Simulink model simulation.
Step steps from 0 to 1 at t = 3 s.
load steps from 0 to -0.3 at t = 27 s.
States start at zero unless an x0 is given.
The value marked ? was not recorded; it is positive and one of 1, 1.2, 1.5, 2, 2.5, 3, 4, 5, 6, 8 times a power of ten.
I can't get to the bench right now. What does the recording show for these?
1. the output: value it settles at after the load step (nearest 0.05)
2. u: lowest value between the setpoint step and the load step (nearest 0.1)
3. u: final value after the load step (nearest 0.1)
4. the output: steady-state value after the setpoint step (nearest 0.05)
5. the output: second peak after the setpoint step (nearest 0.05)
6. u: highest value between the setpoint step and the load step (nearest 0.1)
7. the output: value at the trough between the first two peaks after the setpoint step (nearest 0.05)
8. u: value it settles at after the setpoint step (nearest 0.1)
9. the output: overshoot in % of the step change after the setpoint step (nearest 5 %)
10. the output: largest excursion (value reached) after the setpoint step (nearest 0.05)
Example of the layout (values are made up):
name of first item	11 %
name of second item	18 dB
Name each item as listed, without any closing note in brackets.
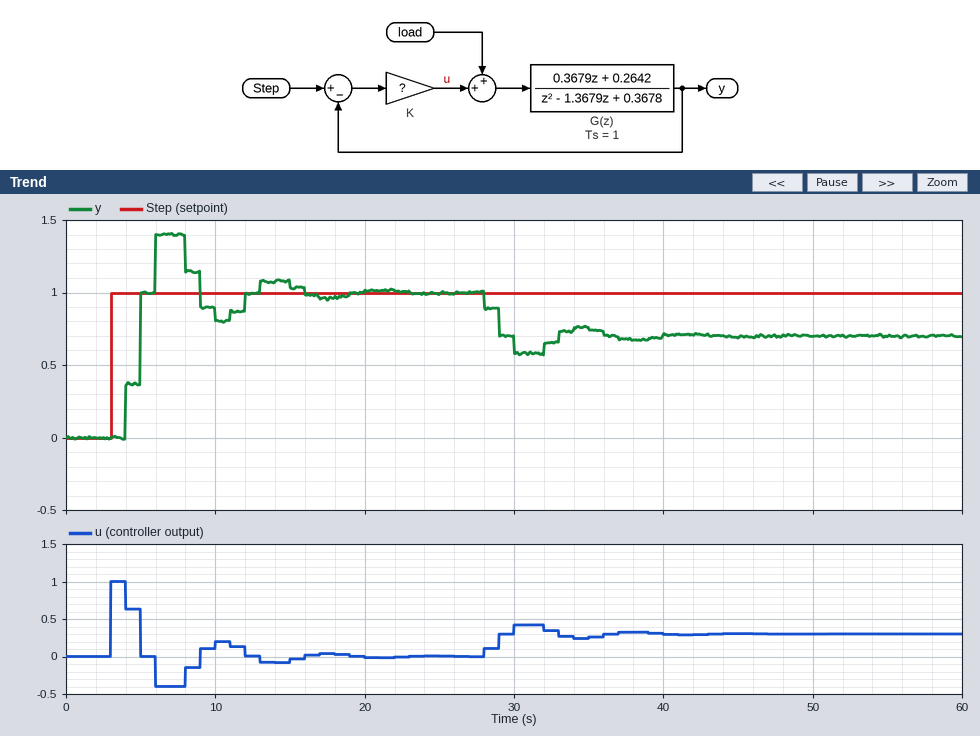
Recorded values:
the output: value it settles at after the load step	0.70
u: lowest value between the setpoint step and the load step	-0.4
u: final value after the load step	0.3
the output: steady-state value after the setpoint step	1.00
the output: second peak after the setpoint step	1.10
u: highest value between the setpoint step and the load step	1.0
the output: value at the trough between the first two peaks after the setpoint step	0.80
u: value it settles at after the setpoint step	0.0
the output: overshoot in % of the step change after the setpoint step	40 %
the output: largest excursion (value reached) after the setpoint step	1.40
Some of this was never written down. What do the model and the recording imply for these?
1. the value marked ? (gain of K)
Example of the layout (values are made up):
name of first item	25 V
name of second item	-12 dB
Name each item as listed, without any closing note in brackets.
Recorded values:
the value marked ?	1
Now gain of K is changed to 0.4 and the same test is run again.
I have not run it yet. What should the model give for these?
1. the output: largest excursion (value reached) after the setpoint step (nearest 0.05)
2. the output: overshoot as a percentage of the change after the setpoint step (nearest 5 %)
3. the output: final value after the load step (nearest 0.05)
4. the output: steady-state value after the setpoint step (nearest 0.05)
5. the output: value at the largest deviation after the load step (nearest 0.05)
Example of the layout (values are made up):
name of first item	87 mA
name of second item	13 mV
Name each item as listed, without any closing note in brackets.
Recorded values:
the output: largest excursion (value reached) after the setpoint step	1.10
the output: overshoot as a percentage of the change after the setpoint step	10 %
the output: final value after the load step	0.25
the output: steady-state value after the setpoint step	1.00
the output: value at the largest deviation after the load step	0.20
